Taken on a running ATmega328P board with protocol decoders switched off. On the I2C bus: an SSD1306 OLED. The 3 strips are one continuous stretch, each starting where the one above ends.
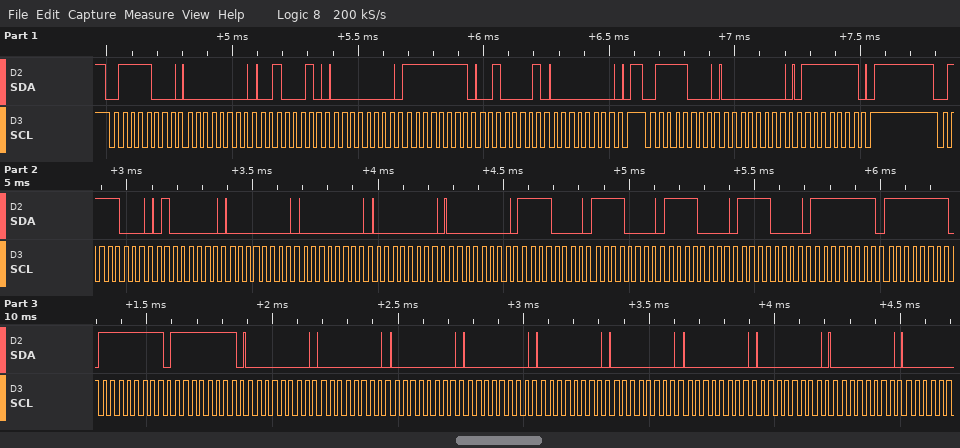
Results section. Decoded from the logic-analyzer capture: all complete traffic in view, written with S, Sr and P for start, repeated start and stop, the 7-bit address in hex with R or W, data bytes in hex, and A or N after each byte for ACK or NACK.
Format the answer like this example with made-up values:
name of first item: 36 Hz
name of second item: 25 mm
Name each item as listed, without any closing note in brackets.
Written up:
all complete traffic in view, written with S, Sr and P for start, repeated start and stop, the 7-bit address in hex with R or W, data bytes in hex, and A or N after each byte for ACK or NACK: S 3CW A 00 A 22 A 00 A FF A 21 A 00 A P S 3CW A 00 A 7F A P S 3CW A 40 A 00 A 00 A 00 A 00 A F0 A F0 A F0 A F0 A FF A FF A FF A FF A 00 A 00 A 00 A 00 A 00 A 00 A 00 A 00 A 00 A
